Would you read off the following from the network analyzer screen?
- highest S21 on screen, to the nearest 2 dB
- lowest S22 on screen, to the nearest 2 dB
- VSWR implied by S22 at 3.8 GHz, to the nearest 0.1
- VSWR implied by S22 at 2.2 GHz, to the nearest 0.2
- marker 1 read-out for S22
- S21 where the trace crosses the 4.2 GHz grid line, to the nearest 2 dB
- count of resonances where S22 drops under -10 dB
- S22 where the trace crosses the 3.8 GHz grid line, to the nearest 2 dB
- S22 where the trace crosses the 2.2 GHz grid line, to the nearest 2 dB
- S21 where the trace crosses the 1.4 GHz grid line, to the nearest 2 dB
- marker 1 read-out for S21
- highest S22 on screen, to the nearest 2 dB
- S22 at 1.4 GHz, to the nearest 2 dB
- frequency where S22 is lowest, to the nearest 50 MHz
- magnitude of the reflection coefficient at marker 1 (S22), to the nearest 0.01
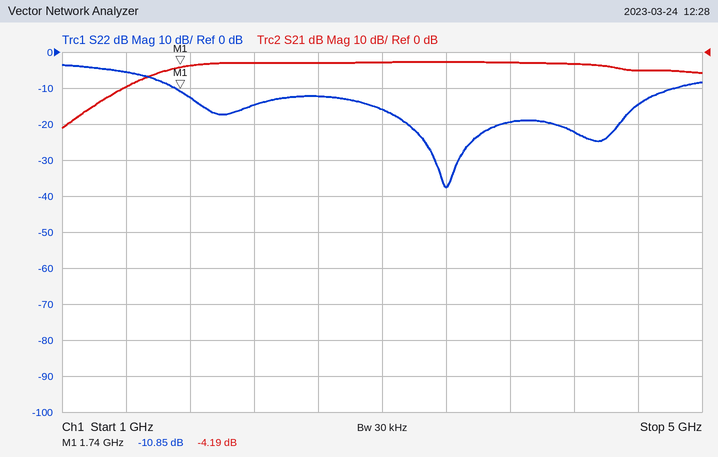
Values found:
-2 dB
-38 dB
1.2
1.4
-10.85 dB
-4 dB
3
-20 dB
-14 dB
-10 dB
-4.19 dB
-4 dB
-6 dB
3.40 GHz
0.29
